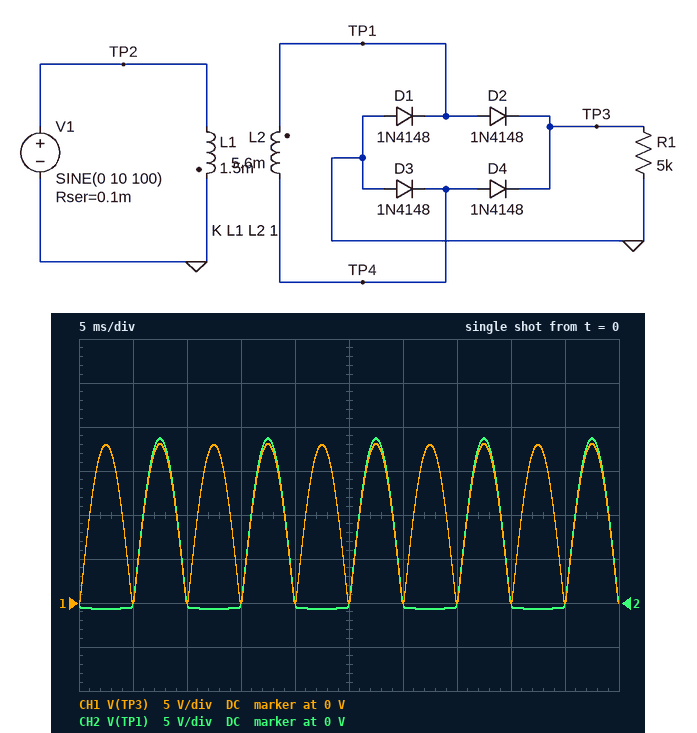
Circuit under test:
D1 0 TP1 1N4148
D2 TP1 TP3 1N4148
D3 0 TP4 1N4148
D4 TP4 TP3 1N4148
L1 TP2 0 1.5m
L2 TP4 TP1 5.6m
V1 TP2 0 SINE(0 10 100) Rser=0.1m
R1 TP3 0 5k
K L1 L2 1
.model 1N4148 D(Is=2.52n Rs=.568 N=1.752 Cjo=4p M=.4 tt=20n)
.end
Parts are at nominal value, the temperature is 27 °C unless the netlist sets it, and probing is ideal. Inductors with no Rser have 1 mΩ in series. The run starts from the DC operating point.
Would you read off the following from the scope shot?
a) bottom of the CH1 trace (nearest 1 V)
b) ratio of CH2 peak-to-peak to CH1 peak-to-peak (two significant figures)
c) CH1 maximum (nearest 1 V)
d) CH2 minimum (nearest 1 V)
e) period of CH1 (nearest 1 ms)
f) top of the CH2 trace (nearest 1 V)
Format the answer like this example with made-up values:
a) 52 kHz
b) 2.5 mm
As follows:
a) 0 V
b) 1.1
c) 18 V
d) -1 V
e) 5 ms
f) 19 V
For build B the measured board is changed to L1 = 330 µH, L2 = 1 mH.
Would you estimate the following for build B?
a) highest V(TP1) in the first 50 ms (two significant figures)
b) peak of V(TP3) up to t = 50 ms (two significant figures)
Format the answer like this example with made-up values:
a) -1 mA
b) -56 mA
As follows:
a) 17 V
b) 16 V
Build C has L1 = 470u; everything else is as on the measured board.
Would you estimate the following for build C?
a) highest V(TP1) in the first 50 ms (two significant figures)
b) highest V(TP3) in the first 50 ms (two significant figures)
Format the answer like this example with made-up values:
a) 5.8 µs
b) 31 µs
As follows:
a) 34 V
b) 33 V
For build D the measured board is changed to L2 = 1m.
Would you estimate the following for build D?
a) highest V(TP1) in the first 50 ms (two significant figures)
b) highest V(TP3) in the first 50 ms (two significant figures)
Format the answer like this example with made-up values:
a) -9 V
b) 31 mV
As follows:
a) 7.6 V
b) 7.0 V
